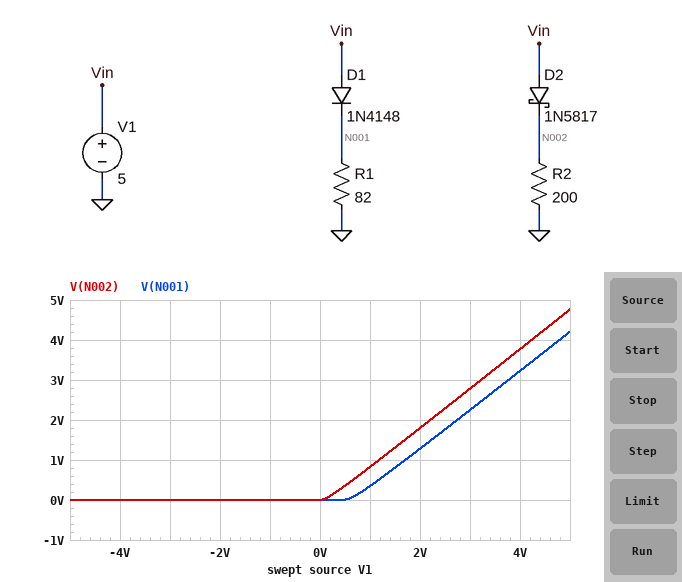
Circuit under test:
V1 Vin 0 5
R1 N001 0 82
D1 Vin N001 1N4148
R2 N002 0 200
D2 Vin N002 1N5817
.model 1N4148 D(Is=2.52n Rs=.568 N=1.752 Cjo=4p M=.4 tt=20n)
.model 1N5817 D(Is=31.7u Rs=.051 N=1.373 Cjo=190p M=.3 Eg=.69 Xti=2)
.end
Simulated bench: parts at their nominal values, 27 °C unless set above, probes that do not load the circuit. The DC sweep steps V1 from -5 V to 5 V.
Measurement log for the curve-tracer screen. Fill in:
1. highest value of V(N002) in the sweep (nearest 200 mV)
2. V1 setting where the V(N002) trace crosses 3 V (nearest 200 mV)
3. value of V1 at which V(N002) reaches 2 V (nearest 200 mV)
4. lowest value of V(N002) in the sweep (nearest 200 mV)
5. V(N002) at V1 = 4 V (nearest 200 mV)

4.8 V
3.2 V
2.2 V
0 V
3.8 V
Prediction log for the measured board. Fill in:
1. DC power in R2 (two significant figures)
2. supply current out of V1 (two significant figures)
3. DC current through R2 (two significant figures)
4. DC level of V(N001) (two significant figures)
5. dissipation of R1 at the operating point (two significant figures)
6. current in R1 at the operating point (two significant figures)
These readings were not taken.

110 mW
75 mA
24 mA
4.2 V
220 mW
51 mA
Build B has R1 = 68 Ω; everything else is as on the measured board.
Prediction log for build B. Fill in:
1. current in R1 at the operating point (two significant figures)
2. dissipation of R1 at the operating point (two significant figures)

62 mA
260 mW
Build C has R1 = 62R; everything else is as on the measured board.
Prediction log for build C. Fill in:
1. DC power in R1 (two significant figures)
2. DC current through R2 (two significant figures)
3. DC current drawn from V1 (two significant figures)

280 mW
24 mA
91 mA
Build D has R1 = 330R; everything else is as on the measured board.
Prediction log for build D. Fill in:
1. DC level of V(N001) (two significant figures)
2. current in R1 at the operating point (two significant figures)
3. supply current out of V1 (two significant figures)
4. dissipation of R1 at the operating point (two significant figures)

4.3 V
13 mA
37 mA
56 mW
